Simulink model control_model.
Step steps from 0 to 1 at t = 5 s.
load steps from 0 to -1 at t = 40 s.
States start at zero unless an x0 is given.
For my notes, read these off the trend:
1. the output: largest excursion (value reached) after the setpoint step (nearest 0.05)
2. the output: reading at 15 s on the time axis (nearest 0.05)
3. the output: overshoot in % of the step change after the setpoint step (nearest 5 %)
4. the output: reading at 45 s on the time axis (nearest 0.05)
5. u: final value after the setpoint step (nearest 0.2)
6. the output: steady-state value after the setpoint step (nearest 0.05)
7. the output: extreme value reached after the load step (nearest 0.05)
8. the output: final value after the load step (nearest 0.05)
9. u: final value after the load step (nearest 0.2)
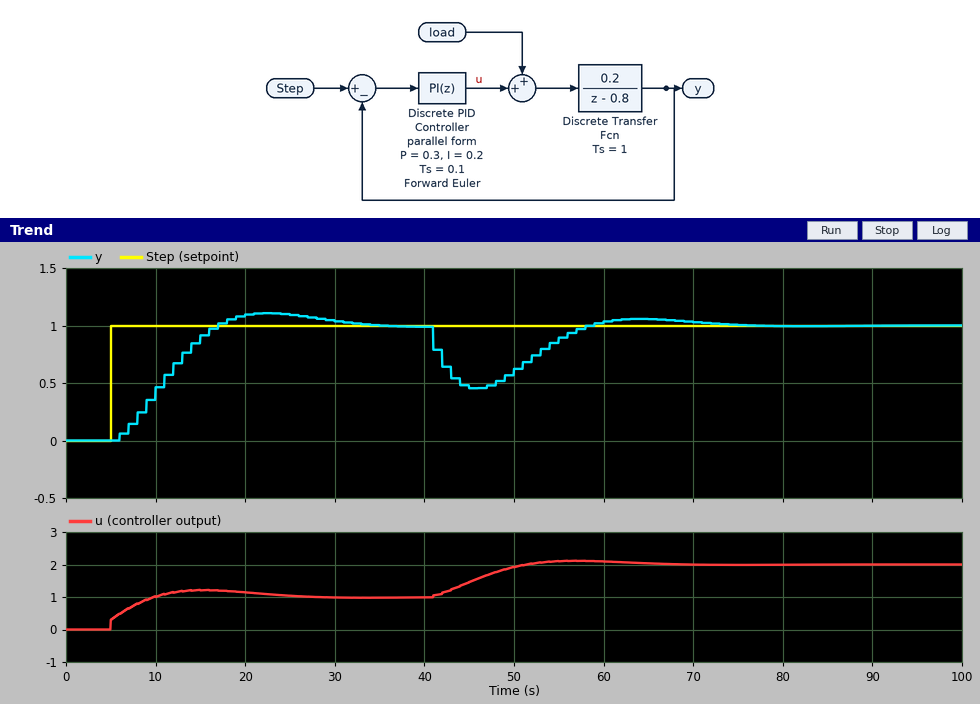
1.10
0.90
10 %
0.45
1.0
1.00
0.45
1.00
2.0
